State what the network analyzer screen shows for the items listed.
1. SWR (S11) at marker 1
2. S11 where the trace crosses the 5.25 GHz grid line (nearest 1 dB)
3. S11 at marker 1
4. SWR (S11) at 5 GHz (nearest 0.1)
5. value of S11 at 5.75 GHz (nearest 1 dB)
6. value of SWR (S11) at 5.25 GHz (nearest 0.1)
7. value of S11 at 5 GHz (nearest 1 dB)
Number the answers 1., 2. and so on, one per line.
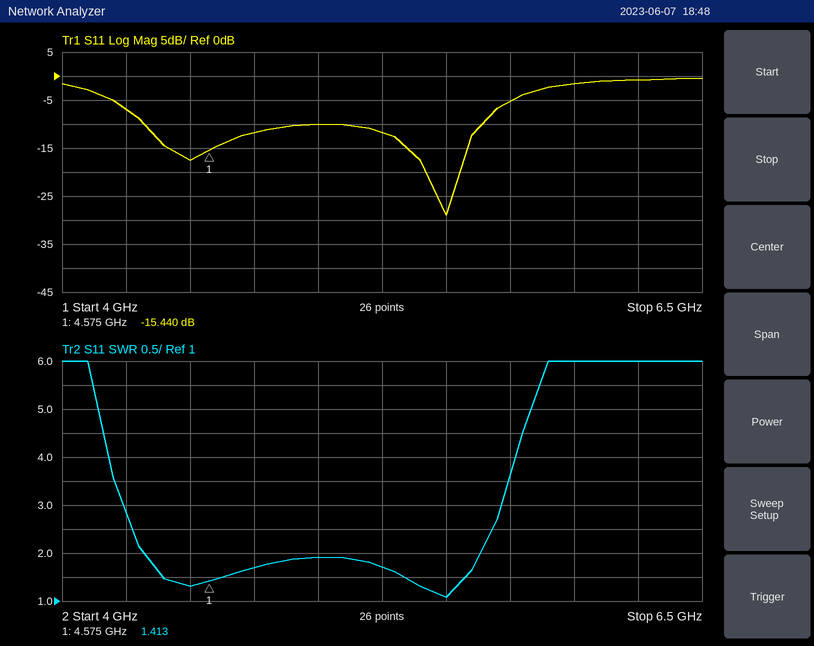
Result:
1. 1.413
2. -12 dB
3. -15.440 dB
4. 1.9
5. -5 dB
6. 1.7
7. -10 dB
